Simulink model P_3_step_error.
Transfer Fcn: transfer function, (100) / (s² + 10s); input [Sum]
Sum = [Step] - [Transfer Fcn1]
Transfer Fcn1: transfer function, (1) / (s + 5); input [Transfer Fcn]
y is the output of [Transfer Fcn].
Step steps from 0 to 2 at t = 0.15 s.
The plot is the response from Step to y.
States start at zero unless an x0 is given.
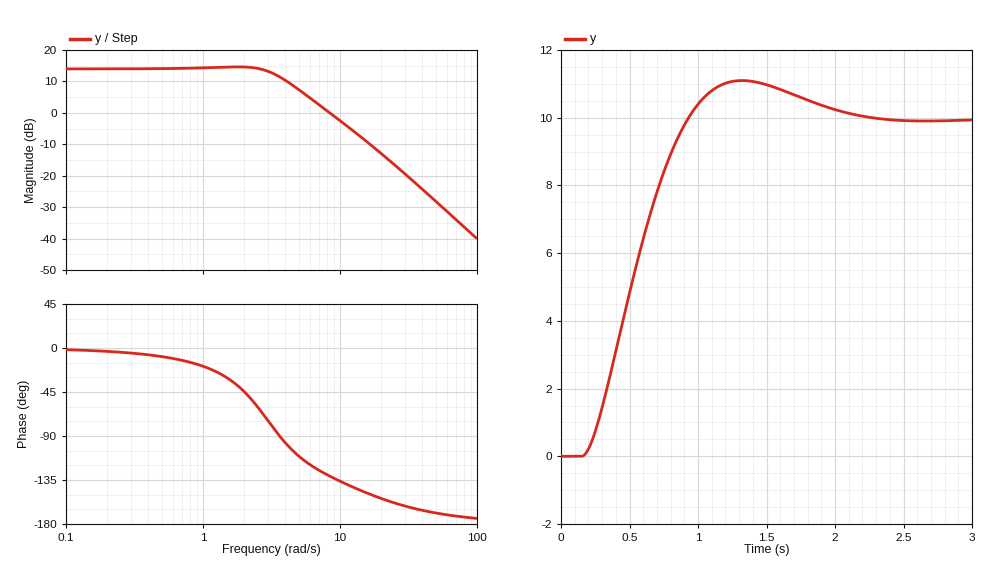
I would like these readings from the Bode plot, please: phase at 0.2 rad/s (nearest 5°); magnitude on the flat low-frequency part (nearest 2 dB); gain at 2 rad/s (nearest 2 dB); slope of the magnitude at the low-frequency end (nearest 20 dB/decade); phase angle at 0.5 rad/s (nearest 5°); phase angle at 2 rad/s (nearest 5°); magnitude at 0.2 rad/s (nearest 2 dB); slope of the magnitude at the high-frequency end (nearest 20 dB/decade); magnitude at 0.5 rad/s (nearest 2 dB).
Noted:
-5°
14 dB
14 dB
0 dB/decade
-10°
-45°
14 dB
-40 dB/decade
14 dB
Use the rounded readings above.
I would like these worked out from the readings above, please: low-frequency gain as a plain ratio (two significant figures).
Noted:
5.0
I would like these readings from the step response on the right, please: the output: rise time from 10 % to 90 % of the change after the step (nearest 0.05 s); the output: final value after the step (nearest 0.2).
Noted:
0.55 s
10.0
